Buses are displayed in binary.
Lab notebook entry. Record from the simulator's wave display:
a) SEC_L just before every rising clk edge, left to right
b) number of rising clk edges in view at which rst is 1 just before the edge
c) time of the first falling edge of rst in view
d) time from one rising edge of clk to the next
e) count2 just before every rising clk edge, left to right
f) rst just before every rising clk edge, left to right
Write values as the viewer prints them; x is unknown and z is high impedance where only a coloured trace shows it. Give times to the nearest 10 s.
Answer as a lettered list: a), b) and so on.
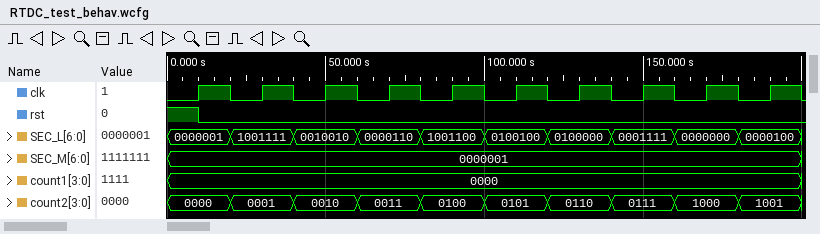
a) 0000001, 1001111, 0010010, 0000110, 1001100, 0100100, 0100000, 0001111, 0000000, 0000100
b) 1
c) 10 s
d) 20 s
e) 0000, 0001, 0010, 0011, 0100, 0101, 0110, 0111, 1000, 1001
f) 1 0 0 0 0 0 0 0 0 0
